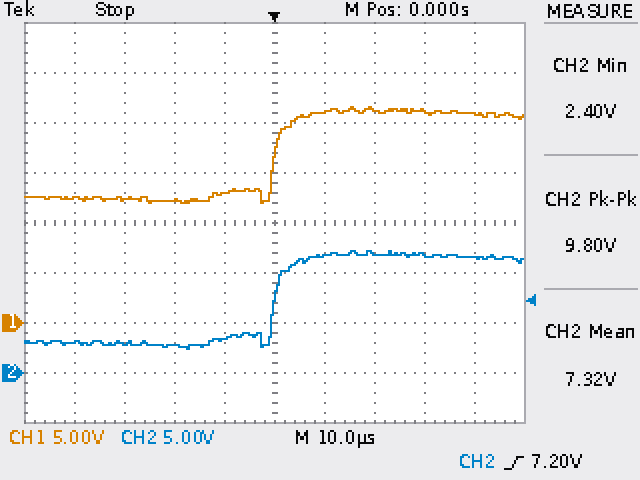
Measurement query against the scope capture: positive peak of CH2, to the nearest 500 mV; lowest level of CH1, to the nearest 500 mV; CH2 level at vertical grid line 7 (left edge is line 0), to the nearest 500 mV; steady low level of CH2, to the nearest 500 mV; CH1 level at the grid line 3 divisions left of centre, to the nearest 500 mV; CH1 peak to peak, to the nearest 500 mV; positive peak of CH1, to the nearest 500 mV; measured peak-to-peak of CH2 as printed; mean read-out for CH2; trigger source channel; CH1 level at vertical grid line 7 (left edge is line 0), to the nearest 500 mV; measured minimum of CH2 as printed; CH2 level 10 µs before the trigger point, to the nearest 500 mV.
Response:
12.0 V
12.0 V
12.0 V
3.0 V
12.5 V
9.5 V
21.5 V
9.80 V
7.32 V
CH2
21.5 V
2.40 V
3.5 V
